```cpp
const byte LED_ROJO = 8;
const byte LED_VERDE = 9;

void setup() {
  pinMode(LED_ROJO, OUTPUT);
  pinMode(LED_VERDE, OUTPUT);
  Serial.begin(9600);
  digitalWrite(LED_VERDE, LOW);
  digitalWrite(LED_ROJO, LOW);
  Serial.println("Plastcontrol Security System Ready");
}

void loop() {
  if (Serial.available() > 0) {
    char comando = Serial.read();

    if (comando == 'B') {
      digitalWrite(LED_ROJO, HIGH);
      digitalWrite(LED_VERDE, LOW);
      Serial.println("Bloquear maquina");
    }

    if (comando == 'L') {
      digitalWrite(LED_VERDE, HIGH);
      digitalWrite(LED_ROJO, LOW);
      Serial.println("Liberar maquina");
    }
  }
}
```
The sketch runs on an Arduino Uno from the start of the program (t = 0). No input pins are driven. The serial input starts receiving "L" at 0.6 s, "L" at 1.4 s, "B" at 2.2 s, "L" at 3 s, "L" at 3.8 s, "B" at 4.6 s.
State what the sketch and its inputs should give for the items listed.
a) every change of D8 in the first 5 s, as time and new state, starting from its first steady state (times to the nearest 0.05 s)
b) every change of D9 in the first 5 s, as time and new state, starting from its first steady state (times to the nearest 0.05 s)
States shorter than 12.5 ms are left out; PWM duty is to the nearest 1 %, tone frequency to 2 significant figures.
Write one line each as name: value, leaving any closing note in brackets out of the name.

every change of D8 in the first 5 s, as time and new state, starting from its first steady state: 0 s low; 2.2 s high; 3 s low; 4.6 s high
every change of D9 in the first 5 s, as time and new state, starting from its first steady state: 0 s low; 0.6 s high; 2.2 s low; 3 s high; 4.6 s low
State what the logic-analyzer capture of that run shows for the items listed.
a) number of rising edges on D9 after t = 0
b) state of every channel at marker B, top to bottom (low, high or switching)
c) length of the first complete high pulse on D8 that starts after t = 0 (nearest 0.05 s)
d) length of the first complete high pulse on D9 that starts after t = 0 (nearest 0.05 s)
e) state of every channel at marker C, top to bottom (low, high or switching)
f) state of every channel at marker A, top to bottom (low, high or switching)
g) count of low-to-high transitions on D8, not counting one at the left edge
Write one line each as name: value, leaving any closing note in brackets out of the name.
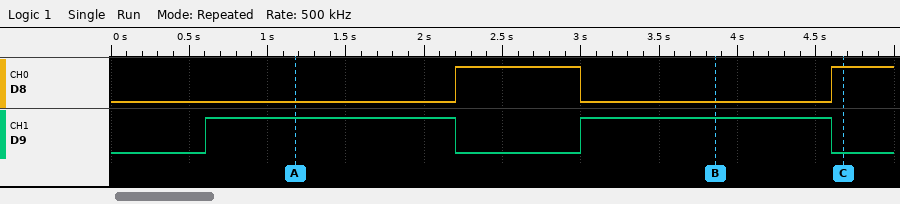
number of rising edges on D9 after t = 0: 2
state of every channel at marker B, top to bottom: D8 low, D9 high
length of the first complete high pulse on D8 that starts after t = 0: 0.80 s
length of the first complete high pulse on D9 that starts after t = 0: 1.60 s
state of every channel at marker C, top to bottom: D8 high, D9 low
state of every channel at marker A, top to bottom: D8 low, D9 high
count of low-to-high transitions on D8, not counting one at the left edge: 2
